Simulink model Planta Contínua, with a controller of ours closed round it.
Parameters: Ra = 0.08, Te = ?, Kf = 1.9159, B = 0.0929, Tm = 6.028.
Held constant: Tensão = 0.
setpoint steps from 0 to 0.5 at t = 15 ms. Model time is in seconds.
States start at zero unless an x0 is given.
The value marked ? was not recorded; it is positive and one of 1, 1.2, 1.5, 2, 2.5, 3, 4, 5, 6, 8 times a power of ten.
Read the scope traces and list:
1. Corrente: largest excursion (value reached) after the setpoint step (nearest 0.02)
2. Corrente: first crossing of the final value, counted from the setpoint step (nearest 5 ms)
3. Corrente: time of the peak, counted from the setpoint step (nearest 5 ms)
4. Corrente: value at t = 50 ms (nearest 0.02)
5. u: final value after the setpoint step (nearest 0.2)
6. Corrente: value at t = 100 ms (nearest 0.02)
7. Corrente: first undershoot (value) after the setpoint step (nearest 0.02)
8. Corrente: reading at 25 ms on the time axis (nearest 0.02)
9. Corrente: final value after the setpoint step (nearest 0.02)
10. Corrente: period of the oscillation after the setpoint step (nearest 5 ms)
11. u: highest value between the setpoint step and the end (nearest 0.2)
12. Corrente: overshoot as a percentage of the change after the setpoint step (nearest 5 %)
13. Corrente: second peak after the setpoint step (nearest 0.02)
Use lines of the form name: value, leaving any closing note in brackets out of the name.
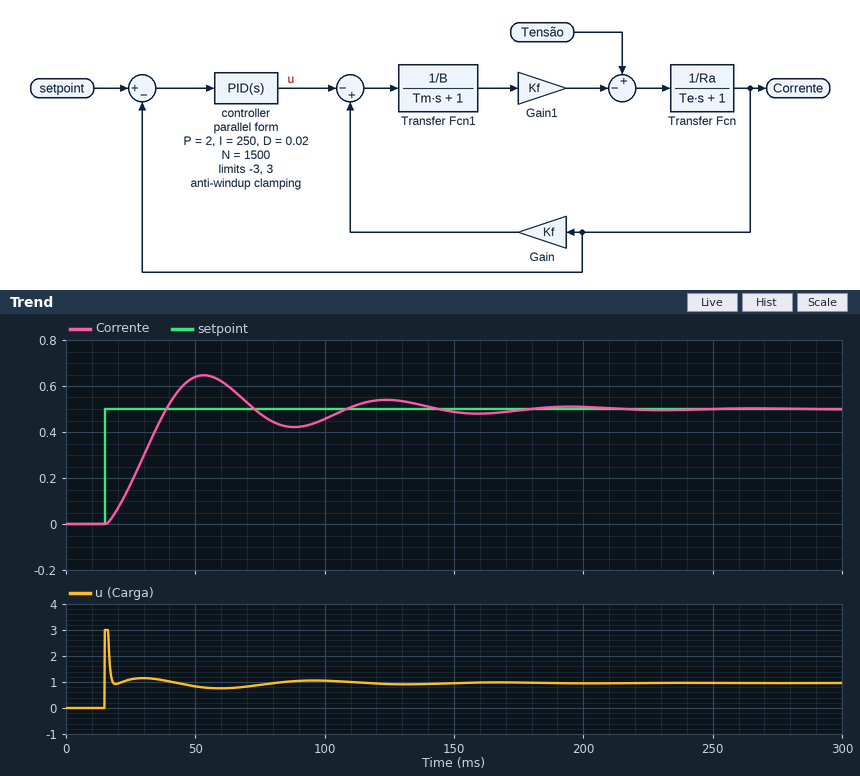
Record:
Corrente: largest excursion (value reached) after the setpoint step: 0.64
Corrente: first crossing of the final value, counted from the setpoint step: 25 ms
Corrente: time of the peak, counted from the setpoint step: 40 ms
Corrente: value at t = 50 ms: 0.64
u: final value after the setpoint step: 1.0
Corrente: value at t = 100 ms: 0.46
Corrente: first undershoot (value) after the setpoint step: 0.42
Corrente: reading at 25 ms on the time axis: 0.18
Corrente: final value after the setpoint step: 0.50
Corrente: period of the oscillation after the setpoint step: 70 ms
u: highest value between the setpoint step and the end: 3.0
Corrente: overshoot as a percentage of the change after the setpoint step: 30 %
Corrente: second peak after the setpoint step: 0.54
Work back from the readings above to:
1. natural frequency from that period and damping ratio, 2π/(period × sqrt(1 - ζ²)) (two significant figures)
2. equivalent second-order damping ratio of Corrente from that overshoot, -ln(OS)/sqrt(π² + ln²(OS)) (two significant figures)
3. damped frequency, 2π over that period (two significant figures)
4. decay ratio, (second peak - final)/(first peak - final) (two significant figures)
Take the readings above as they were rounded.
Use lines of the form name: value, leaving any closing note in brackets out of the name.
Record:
natural frequency from that period and damping ratio, 2π/(period × sqrt(1 - ζ²)): 0.096 rad/ms
equivalent second-order damping ratio of Corrente from that overshoot, -ln(OS)/sqrt(π² + ln²(OS)): 0.36
damped frequency, 2π over that period: 0.090 rad/ms
decay ratio, (second peak - final)/(first peak - final): 0.29
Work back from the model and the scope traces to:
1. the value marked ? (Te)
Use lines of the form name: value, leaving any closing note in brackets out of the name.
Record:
the value marked ?: 0.015
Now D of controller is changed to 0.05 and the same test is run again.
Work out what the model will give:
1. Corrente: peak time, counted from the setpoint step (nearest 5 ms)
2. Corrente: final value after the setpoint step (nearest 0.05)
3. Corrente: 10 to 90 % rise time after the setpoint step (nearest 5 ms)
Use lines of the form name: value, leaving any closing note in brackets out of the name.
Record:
Corrente: peak time, counted from the setpoint step: 50 ms
Corrente: final value after the setpoint step: 0.50
Corrente: 10 to 90 % rise time after the setpoint step: 25 ms
